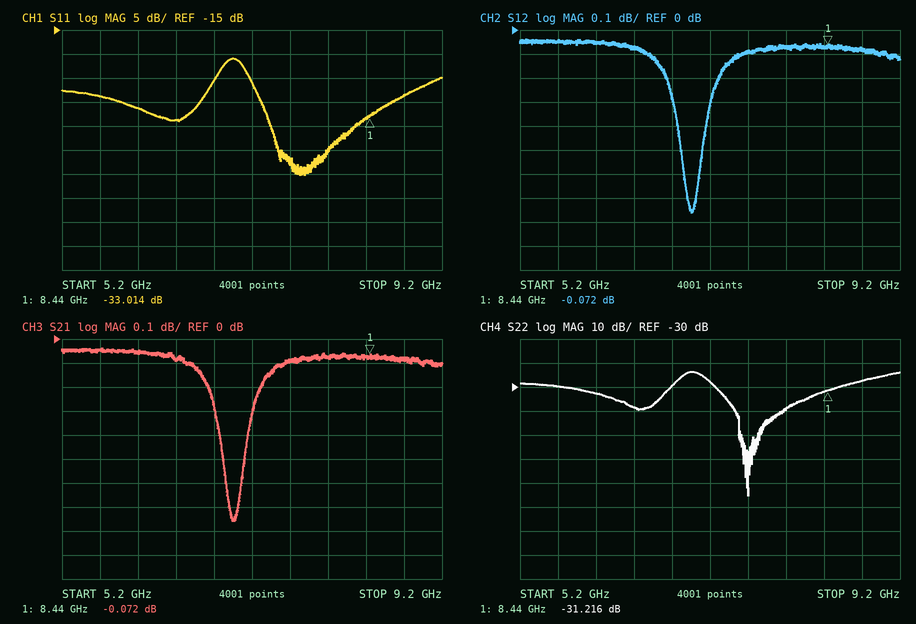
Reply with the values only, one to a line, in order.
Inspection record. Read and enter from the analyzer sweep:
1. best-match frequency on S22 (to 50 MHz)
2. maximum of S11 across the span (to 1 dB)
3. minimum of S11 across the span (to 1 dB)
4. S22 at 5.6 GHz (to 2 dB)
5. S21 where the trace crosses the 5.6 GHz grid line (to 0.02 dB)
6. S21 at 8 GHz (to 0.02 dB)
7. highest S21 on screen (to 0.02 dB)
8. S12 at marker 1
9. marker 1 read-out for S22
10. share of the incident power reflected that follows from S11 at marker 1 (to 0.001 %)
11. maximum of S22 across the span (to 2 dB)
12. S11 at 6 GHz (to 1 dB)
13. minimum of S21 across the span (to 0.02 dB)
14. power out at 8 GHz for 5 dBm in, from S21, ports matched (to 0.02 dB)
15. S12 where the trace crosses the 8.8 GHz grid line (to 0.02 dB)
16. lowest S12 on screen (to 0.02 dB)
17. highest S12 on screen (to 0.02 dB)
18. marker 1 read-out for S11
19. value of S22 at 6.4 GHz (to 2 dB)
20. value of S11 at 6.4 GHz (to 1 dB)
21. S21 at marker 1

7.60 GHz
-21 dB
-45 dB
-30 dB
-0.04 dB
-0.08 dB
-0.04 dB
-0.072 dB
-31.216 dB
0.050 %
-24 dB
-31 dB
-0.76 dB
4.92 dBm
-0.08 dB
-0.76 dB
-0.04 dB
-33.014 dB
-38 dB
-34 dB
-0.072 dB
